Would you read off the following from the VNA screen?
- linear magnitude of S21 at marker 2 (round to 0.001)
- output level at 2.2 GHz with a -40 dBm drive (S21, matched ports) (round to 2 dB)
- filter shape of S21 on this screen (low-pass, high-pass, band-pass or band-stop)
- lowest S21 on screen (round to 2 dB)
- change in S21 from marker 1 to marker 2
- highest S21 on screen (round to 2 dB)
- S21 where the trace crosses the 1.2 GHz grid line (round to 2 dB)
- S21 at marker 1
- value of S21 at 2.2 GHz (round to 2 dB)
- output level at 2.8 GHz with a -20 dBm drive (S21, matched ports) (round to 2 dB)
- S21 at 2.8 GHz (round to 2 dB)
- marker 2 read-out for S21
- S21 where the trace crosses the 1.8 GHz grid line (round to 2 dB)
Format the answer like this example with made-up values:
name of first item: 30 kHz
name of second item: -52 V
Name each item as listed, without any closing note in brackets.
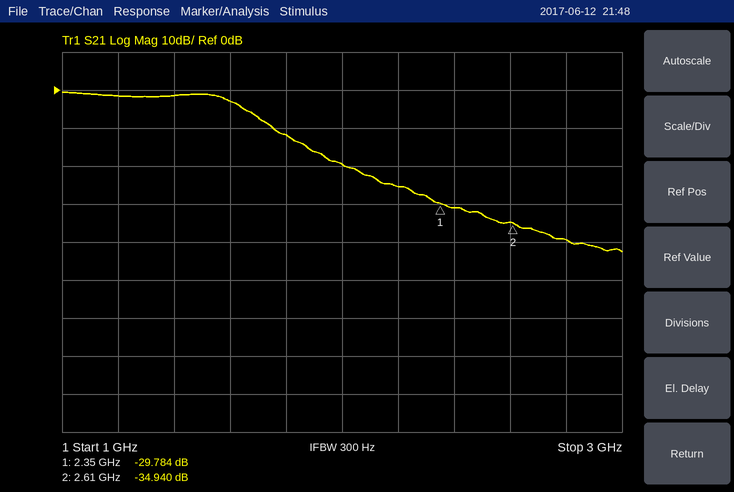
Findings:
linear magnitude of S21 at marker 2: 0.018
output level at 2.2 GHz with a -40 dBm drive (S21, matched ports): -66 dBm
filter shape of S21 on this screen: low-pass
lowest S21 on screen: -42 dB
change in S21 from marker 1 to marker 2: -5.156 dB
highest S21 on screen: 0 dB
S21 where the trace crosses the 1.2 GHz grid line: -2 dB
S21 at marker 1: -29.784 dB
value of S21 at 2.2 GHz: -26 dB
output level at 2.8 GHz with a -20 dBm drive (S21, matched ports): -60 dBm
S21 at 2.8 GHz: -40 dB
marker 2 read-out for S21: -34.940 dB
S21 where the trace crosses the 1.8 GHz grid line: -12 dB
